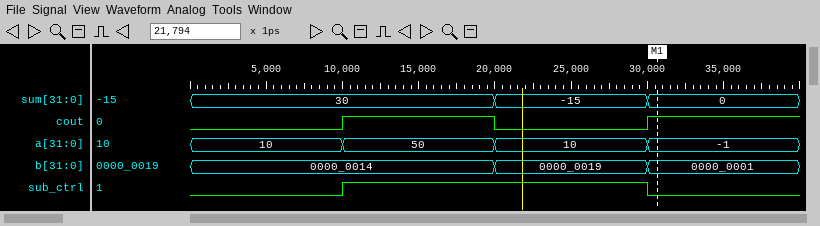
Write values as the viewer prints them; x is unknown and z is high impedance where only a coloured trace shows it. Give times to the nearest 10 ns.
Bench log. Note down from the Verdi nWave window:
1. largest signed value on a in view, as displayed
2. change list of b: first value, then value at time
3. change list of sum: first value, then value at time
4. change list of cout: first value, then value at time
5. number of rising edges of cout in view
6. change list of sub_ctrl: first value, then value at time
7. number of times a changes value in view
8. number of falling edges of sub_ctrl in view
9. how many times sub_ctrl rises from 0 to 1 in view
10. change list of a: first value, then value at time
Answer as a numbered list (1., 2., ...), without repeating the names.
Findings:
1. 50
2. 0000_0014, 0000_0019 at 20 ns, 0000_0001 at 30 ns
3. 30, -15 at 20 ns, 0 at 30 ns
4. 0, 1 at 10 ns, 0 at 20 ns, 1 at 30 ns
5. 2
6. 0, 1 at 10 ns, 0 at 30 ns
7. 3
8. 1
9. 1
10. 10, 50 at 10 ns, 10 at 20 ns, -1 at 30 ns
